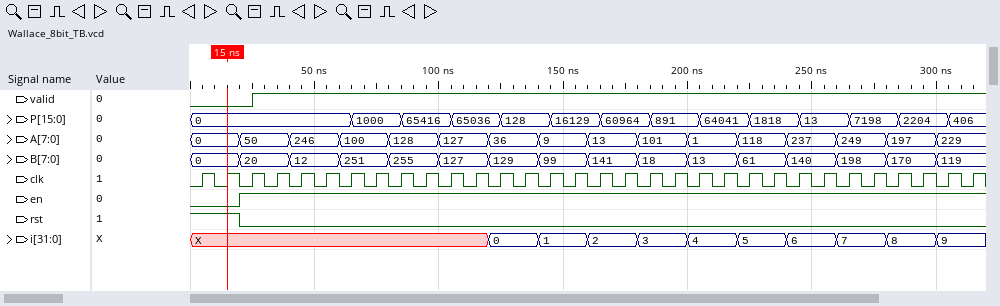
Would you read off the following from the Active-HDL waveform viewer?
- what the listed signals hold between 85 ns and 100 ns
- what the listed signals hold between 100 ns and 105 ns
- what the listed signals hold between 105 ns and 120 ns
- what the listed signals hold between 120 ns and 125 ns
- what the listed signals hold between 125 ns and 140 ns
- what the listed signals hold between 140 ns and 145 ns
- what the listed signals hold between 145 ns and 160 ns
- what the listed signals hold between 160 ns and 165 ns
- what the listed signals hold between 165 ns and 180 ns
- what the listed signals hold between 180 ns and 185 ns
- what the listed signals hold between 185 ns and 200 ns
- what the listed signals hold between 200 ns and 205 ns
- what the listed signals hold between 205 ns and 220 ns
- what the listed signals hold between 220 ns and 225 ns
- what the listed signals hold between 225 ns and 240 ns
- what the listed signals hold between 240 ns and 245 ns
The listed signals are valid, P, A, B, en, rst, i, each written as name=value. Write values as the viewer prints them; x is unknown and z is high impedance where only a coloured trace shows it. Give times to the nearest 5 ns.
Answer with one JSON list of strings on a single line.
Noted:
["valid=1, P=65416, A=128, B=255, en=1, rst=0, i=X", "valid=1, P=65416, A=127, B=127, en=1, rst=0, i=X", "valid=1, P=65036, A=127, B=127, en=1, rst=0, i=X", "valid=1, P=65036, A=36, B=129, en=1, rst=0, i=0", "valid=1, P=128, A=36, B=129, en=1, rst=0, i=0", "valid=1, P=128, A=9, B=99, en=1, rst=0, i=1", "valid=1, P=16129, A=9, B=99, en=1, rst=0, i=1", "valid=1, P=16129, A=13, B=141, en=1, rst=0, i=2", "valid=1, P=60964, A=13, B=141, en=1, rst=0, i=2", "valid=1, P=60964, A=101, B=18, en=1, rst=0, i=3", "valid=1, P=891, A=101, B=18, en=1, rst=0, i=3", "valid=1, P=891, A=1, B=13, en=1, rst=0, i=4", "valid=1, P=64041, A=1, B=13, en=1, rst=0, i=4", "valid=1, P=64041, A=118, B=61, en=1, rst=0, i=5", "valid=1, P=1818, A=118, B=61, en=1, rst=0, i=5", "valid=1, P=1818, A=237, B=140, en=1, rst=0, i=6"]
